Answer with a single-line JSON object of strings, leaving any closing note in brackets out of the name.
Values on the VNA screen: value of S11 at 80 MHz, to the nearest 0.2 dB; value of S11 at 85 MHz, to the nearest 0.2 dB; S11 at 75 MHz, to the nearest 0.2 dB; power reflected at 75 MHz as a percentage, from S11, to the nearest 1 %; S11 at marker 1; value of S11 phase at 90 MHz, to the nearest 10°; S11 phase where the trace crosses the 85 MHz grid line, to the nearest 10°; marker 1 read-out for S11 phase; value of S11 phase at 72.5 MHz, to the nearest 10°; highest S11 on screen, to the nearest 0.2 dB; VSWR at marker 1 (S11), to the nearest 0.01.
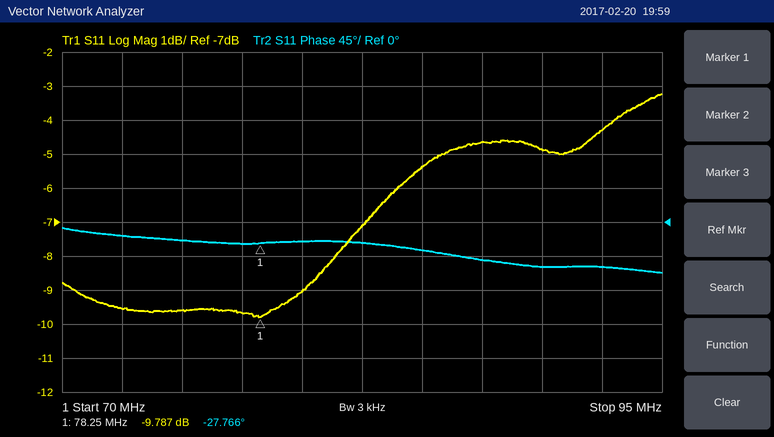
{"value of S11 at 80 MHz, to the nearest 0.2 dB": "-9.0 dB", "value of S11 at 85 MHz, to the nearest 0.2 dB": "-5.4 dB", "S11 at 75 MHz, to the nearest 0.2 dB": "-9.6 dB", "power reflected at 75 MHz as a percentage, from S11, to the nearest 1 %": "11 %", "S11 at marker 1": "-9.787 dB", "value of S11 phase at 90 MHz, to the nearest 10°": "-60°", "S11 phase where the trace crosses the 85 MHz grid line, to the nearest 10°": "-40°", "marker 1 read-out for S11 phase": "-27.766°", "value of S11 phase at 72.5 MHz, to the nearest 10°": "-20°", "highest S11 on screen, to the nearest 0.2 dB": "-3.2 dB", "VSWR at marker 1 (S11), to the nearest 0.01": "1.96"}
